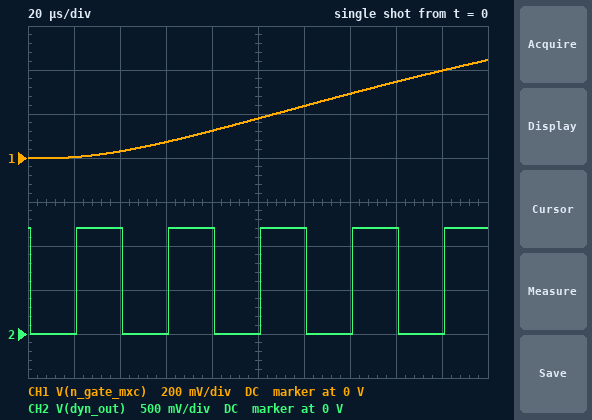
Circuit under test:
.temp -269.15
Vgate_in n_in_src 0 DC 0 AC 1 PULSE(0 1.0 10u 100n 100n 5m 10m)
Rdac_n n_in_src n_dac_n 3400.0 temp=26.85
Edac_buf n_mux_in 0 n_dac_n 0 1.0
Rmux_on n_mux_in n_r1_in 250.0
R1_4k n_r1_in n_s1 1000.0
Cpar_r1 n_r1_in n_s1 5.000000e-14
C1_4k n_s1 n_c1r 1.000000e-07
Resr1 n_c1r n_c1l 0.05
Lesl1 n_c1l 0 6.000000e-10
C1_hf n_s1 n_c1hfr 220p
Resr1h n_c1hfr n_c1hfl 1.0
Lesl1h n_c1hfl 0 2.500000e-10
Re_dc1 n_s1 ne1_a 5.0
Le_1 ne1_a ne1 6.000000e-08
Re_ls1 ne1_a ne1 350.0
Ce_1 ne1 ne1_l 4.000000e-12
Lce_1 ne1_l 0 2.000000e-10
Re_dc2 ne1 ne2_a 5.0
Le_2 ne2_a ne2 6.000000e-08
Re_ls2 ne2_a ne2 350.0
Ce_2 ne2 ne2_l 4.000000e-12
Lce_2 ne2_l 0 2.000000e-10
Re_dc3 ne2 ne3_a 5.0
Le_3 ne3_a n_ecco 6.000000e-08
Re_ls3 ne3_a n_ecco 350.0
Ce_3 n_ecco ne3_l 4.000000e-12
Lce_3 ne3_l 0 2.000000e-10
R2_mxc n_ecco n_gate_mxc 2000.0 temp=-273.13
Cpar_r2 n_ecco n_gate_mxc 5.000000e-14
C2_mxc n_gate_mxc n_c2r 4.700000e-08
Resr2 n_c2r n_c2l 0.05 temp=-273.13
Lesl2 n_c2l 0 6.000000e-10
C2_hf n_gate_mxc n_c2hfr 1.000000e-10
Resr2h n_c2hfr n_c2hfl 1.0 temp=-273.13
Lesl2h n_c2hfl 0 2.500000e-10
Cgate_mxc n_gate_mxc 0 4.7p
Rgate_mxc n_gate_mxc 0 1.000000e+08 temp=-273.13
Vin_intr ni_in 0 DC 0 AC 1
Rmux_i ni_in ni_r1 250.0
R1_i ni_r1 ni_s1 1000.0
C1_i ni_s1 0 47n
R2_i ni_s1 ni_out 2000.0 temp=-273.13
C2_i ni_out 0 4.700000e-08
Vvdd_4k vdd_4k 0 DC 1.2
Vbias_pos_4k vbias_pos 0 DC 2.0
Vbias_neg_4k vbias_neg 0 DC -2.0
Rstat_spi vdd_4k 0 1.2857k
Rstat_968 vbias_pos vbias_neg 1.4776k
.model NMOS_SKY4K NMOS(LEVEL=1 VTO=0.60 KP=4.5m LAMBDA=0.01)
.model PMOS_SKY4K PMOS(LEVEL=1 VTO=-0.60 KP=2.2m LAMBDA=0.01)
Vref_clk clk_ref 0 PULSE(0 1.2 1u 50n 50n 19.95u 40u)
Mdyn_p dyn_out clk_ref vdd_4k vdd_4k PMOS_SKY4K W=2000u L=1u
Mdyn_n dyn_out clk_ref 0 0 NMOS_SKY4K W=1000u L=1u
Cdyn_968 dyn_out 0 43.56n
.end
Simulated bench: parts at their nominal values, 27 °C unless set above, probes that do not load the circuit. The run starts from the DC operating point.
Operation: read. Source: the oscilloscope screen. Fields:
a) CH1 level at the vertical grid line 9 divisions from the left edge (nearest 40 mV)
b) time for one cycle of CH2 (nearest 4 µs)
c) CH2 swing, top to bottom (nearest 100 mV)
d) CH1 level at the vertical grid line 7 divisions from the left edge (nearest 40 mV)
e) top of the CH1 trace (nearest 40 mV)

400 mV
40 µs
1.2 V
280 mV
440 mV
